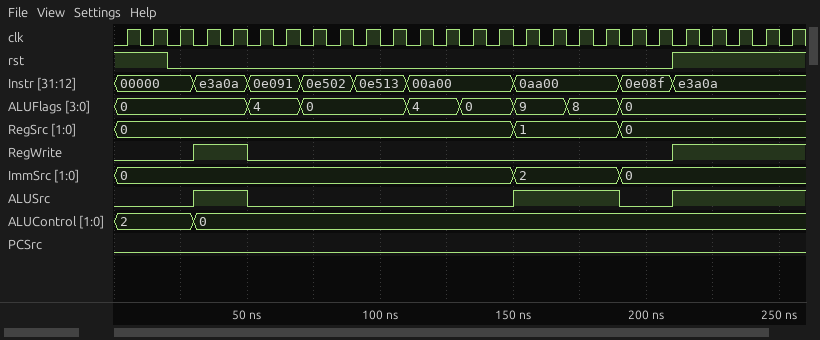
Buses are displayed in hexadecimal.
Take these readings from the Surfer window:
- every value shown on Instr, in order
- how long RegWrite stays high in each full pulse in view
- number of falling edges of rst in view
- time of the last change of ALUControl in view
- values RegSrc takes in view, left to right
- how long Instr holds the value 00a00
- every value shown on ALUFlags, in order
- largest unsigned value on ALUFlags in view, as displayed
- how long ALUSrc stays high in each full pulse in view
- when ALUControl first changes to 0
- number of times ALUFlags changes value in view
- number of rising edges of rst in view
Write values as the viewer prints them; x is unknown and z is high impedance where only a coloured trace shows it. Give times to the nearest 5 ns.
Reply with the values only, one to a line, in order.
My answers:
00000, e3a0a, 0e091, 0e502, 0e513, 00a00, 0aa00, 0e08f, e3a0a
20 ns
1
30 ns
0, 1, 0
40 ns
0, 4, 0, 4, 0, 9, 8, 0
9
20 ns, 40 ns
30 ns
7
1
